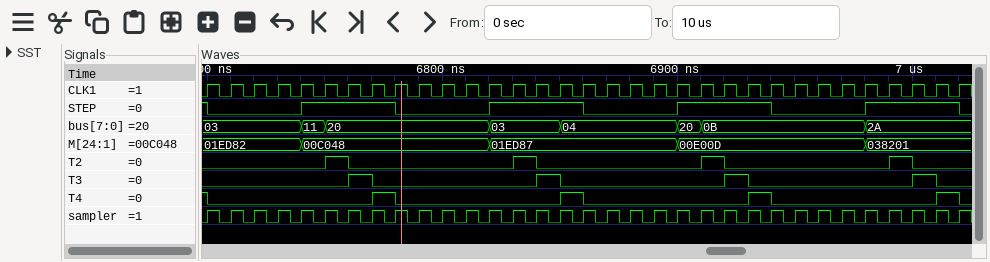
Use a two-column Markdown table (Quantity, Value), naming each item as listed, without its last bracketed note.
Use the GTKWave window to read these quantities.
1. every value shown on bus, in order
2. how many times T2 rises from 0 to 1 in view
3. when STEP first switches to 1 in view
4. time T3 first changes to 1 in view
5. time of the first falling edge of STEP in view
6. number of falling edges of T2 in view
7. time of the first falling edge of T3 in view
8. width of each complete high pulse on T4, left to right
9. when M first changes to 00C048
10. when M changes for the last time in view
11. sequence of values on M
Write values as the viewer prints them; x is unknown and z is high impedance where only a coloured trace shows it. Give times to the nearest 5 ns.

| Quantity | Value |
|---|---|
| every value shown on bus, in order | 03, 11, 20, 03, 04, 20, 0B, 2A |
| how many times T2 rises from 0 to 1 in view | 4 |
| when STEP first switches to 1 in view | 6740 ns |
| time T3 first changes to 1 in view | 6760 ns |
| time of the first falling edge of STEP in view | 6700 ns |
| number of falling edges of T2 in view | 4 |
| time of the first falling edge of T3 in view | 6770 ns |
| width of each complete high pulse on T4, left to right | 10 ns, 10 ns, 10 ns, 10 ns |
| when M first changes to 00C048 | 6740 ns |
| when M changes for the last time in view | 6980 ns |
| sequence of values on M | 01ED82, 00C048, 01ED87, 00E00D, 038201 |
